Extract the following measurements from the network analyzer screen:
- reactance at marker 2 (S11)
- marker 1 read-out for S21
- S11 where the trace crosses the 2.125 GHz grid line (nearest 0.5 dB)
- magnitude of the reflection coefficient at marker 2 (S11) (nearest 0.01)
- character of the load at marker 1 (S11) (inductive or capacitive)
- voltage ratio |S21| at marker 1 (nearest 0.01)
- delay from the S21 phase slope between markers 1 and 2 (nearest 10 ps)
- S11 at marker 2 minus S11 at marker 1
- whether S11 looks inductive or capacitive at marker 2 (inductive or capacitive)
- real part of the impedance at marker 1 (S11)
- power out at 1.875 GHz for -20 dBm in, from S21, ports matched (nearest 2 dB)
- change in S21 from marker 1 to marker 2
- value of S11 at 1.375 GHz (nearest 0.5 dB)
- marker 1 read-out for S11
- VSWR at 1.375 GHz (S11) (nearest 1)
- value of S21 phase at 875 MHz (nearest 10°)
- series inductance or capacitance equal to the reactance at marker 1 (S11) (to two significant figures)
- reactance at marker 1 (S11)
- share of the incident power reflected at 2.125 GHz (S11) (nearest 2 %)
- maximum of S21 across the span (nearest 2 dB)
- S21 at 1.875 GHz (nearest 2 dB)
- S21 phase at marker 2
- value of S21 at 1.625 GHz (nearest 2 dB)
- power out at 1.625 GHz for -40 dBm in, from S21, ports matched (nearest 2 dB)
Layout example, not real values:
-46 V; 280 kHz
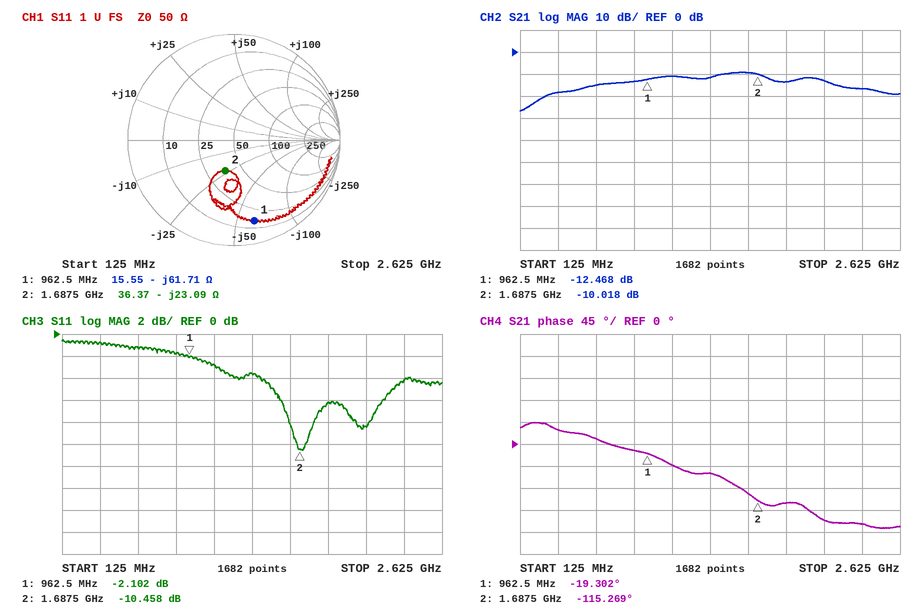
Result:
-23.09 Ω; -12.468 dB; -8.5 dB; 0.30; capacitive; 0.24; 370 ps; -8.356 dB; capacitive; 15.55 Ω; -34 dBm; 2.450 dB; -3.5 dB; -2.102 dB; 5; -10°; 2.7 pF; -61.71 Ω; 14 %; -10 dB; -14 dB; -115.269°; -10 dB; -50 dBm
